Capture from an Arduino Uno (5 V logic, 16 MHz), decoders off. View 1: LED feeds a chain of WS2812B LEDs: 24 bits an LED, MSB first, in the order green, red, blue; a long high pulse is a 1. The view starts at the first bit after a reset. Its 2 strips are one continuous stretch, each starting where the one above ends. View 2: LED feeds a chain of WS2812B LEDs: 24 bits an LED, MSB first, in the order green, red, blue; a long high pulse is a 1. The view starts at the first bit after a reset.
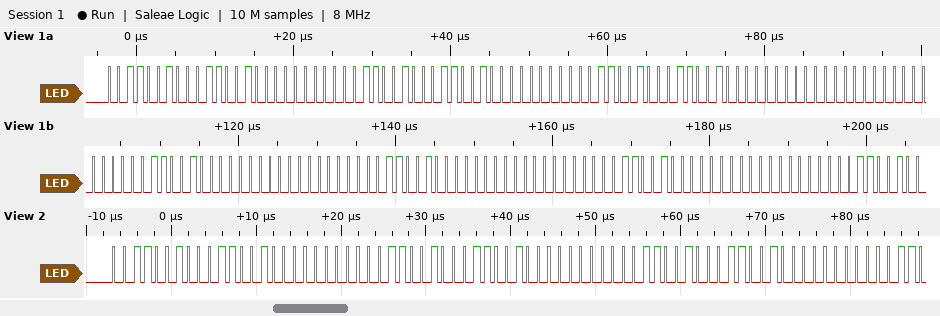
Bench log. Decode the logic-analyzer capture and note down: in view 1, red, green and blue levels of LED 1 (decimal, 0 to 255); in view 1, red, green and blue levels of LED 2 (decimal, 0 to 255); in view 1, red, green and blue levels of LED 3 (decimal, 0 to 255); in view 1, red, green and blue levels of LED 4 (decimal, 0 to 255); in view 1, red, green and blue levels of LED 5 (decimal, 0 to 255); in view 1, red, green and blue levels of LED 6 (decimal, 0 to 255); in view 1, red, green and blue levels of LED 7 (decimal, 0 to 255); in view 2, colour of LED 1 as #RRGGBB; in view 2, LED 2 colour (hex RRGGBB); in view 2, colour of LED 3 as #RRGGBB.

50, 50, 0
50, 50, 0
50, 50, 0
0, 0, 50
0, 0, 50
0, 0, 50
0, 0, 50
#323200
#323200
#323200
